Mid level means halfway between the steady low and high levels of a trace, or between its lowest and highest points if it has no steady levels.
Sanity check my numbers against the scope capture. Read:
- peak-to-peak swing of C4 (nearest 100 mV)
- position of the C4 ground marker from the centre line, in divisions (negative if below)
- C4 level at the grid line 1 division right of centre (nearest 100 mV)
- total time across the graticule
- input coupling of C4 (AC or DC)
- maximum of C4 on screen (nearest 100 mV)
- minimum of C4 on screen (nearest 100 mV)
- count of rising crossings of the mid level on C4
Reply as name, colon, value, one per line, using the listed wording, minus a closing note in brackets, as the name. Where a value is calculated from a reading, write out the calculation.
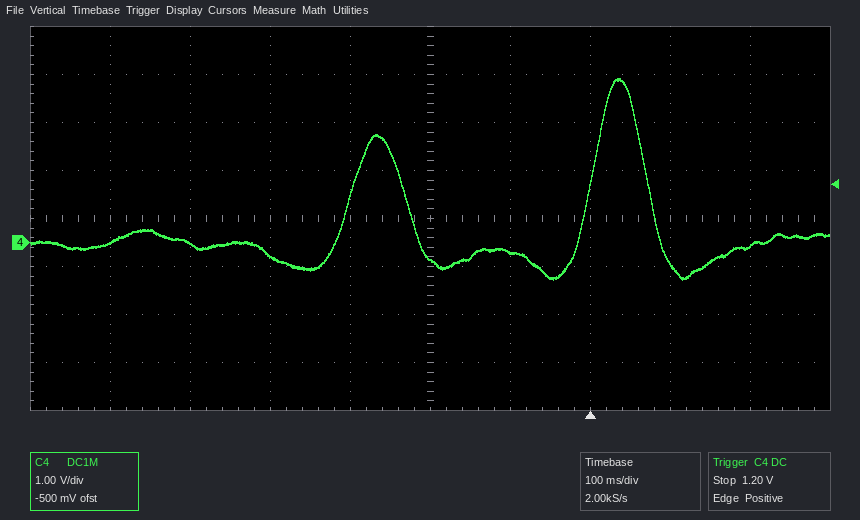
peak-to-peak swing of C4: 3.4 V − (-800 mV) = 4.2 V
position of the C4 ground marker from the centre line, in divisions: -0.5 div
C4 level at the grid line 1 division right of centre: -200 mV
total time across the graticule: 1 s
input coupling of C4: DC
maximum of C4 on screen: 3.4 V
minimum of C4 on screen: -800 mV
count of rising crossings of the mid level on C4: 2
